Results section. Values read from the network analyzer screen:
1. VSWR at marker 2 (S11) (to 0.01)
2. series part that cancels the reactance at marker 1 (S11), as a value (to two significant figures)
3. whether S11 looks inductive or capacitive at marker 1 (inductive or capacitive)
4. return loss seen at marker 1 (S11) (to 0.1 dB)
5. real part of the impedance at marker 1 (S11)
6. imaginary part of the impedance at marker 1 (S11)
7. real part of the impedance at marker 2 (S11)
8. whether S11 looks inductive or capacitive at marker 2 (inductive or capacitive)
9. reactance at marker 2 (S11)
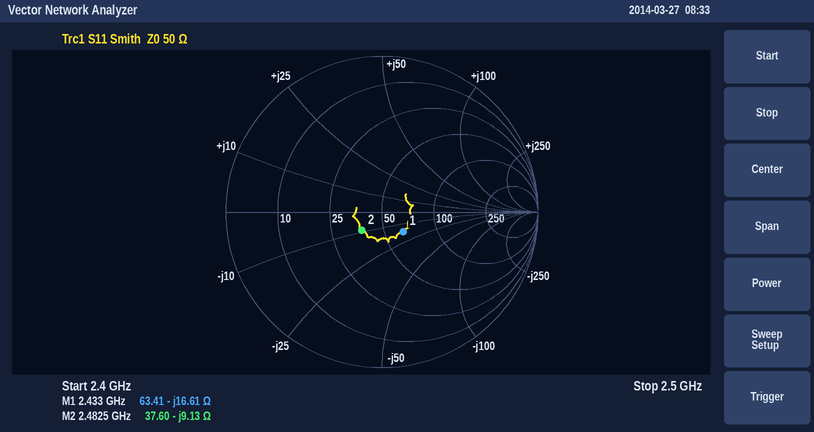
1.42
1.1 nH
capacitive
14.6 dB
63.41 Ω
-16.61 Ω
37.60 Ω
capacitive
-9.13 Ω
